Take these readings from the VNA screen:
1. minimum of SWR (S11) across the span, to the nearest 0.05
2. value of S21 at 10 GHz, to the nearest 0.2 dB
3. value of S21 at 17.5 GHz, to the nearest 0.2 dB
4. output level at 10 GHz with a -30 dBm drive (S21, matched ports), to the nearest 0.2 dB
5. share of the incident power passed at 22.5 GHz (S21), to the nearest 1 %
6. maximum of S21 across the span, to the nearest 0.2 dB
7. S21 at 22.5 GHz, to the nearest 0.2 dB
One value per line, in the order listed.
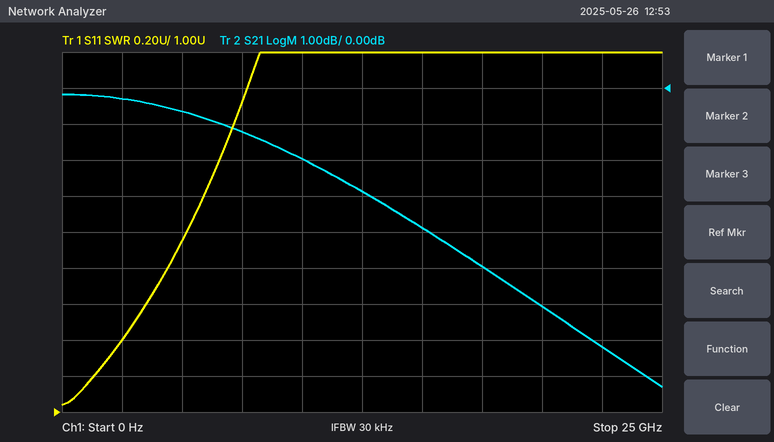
1.05
-2.0 dB
-5.0 dB
-32.0 dBm
19 %
-0.2 dB
-7.2 dB
